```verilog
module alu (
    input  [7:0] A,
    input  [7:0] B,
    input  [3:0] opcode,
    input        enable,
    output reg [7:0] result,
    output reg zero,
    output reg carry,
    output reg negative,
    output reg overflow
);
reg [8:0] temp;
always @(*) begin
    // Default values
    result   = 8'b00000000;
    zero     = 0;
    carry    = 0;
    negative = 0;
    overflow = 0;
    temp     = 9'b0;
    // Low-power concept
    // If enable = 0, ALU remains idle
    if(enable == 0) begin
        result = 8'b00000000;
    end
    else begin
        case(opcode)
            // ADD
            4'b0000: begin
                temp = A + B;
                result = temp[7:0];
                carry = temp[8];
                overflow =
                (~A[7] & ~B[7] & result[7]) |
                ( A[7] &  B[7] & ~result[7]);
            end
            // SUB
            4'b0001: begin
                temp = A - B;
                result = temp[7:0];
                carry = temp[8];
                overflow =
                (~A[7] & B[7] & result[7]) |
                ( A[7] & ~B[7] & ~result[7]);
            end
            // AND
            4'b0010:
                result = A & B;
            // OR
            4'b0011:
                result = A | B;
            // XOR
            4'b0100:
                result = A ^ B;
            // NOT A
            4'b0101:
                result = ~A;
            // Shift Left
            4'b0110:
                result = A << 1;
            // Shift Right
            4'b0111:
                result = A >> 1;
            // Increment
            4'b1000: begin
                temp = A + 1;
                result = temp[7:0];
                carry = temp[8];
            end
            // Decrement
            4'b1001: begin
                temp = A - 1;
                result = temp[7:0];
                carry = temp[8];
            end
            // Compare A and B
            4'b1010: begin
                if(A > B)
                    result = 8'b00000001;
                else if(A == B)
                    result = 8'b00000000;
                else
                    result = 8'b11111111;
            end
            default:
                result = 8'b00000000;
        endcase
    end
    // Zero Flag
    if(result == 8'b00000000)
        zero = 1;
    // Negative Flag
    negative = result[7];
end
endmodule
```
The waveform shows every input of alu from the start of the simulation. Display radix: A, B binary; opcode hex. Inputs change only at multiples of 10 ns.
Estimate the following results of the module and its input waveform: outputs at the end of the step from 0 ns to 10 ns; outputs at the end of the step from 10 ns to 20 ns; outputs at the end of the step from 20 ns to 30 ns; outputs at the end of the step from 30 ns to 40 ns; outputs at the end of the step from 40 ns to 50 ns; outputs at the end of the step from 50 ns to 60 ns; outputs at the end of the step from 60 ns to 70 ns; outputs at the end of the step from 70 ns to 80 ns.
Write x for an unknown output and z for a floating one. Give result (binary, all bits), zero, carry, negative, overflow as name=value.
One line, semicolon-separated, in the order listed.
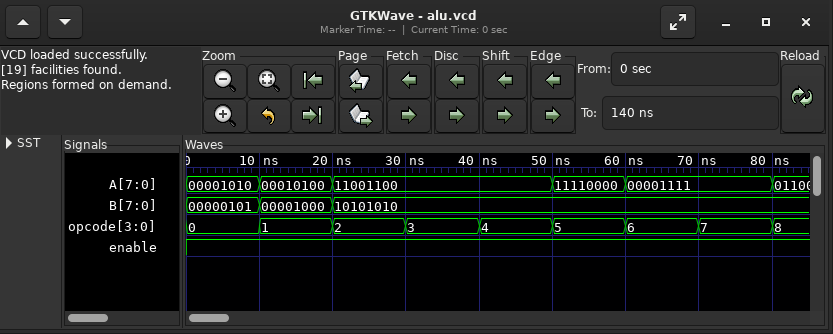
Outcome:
result=00001111, zero=0, carry=0, negative=0, overflow=0; result=00001100, zero=0, carry=0, negative=0, overflow=0; result=10001000, zero=0, carry=0, negative=1, overflow=0; result=11101110, zero=0, carry=0, negative=1, overflow=0; result=01100110, zero=0, carry=0, negative=0, overflow=0; result=00001111, zero=0, carry=0, negative=0, overflow=0; result=00011110, zero=0, carry=0, negative=0, overflow=0; result=00000111, zero=0, carry=0, negative=0, overflow=0
